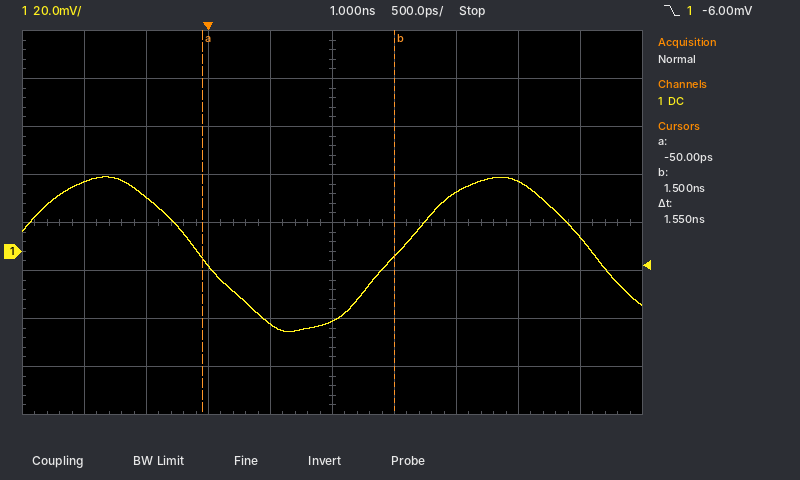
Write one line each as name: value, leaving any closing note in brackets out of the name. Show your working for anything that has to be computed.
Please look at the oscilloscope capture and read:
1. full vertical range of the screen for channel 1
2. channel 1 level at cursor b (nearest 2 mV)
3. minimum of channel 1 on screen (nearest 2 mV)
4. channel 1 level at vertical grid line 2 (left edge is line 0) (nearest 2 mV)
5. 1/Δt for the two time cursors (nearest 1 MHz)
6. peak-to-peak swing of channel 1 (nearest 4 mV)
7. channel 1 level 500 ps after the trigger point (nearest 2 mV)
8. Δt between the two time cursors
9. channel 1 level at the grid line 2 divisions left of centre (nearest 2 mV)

full vertical range of the screen for channel 1: 160 mV
channel 1 level at cursor b: -2 mV
minimum of channel 1 on screen: -34 mV
channel 1 level at vertical grid line 2 (left edge is line 0): 22 mV
1/Δt for the two time cursors: 1 / 1.55 ns ≈ 645 MHz
peak-to-peak swing of channel 1: 64 mV
channel 1 level 500 ps after the trigger point: -30 mV
Δt between the two time cursors: 1.55 ns
channel 1 level at the grid line 2 divisions left of centre: -6 mV
